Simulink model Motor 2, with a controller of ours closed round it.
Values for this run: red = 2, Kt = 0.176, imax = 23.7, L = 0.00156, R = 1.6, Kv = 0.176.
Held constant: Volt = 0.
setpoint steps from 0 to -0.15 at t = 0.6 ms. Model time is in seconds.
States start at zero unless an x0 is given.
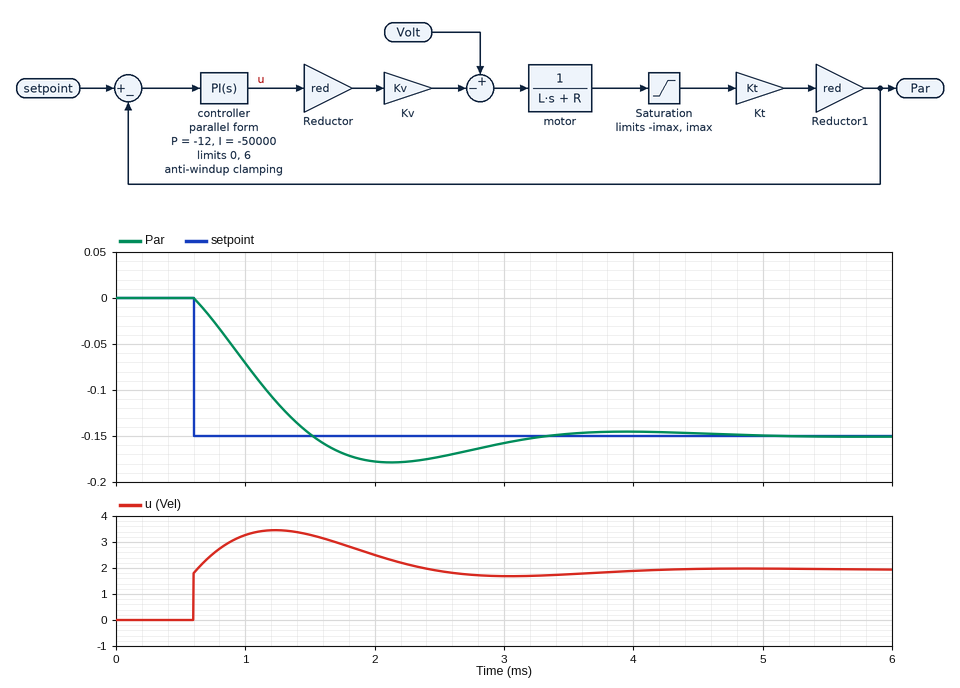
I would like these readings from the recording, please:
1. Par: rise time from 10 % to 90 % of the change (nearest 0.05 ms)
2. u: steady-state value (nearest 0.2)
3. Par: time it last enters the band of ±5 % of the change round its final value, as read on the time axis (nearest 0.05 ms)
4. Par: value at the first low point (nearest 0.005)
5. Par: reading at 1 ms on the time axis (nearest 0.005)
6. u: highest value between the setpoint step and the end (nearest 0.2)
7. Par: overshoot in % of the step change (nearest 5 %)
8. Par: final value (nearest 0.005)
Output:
0.70 ms
2.0
3.00 ms
-0.180
-0.070
3.4
20 %
-0.150
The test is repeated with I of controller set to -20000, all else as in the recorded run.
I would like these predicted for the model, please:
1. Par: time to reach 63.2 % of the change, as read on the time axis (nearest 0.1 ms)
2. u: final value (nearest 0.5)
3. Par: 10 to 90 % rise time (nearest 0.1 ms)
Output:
1.4 ms
2.0
1.4 ms
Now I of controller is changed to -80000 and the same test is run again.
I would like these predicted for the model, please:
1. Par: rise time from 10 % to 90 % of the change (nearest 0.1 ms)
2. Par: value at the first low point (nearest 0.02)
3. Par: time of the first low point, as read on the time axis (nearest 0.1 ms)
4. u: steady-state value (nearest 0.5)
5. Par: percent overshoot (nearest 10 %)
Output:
0.5 ms
-0.20
1.8 ms
2.0
30 %
